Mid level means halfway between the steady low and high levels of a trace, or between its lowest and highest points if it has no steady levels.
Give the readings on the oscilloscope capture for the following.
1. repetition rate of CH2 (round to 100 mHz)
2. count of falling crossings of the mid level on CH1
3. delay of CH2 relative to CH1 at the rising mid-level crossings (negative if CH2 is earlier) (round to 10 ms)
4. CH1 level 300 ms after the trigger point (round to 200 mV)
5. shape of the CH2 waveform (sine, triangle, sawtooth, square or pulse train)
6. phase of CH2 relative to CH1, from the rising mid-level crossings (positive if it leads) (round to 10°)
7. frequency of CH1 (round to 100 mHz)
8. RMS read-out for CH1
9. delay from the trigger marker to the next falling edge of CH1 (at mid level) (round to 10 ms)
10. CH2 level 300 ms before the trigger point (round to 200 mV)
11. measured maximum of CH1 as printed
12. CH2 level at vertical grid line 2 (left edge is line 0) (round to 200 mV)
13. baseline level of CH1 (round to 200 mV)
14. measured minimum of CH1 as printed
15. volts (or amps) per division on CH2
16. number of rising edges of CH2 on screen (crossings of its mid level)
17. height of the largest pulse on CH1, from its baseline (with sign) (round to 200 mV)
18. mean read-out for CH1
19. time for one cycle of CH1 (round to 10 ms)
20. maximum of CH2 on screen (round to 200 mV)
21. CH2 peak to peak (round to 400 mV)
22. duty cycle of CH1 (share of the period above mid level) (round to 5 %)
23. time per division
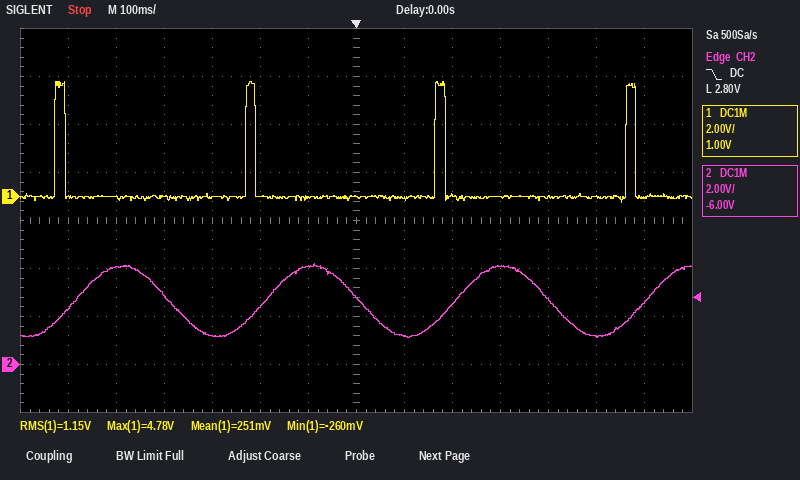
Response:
2.5 Hz
4
+40 ms
0.0 V
sine
-40°
2.5 Hz
1.15 V
190 ms
1.2 V
4.78 V
4.0 V
0.0 V
-260 mV
2 V
4
+4.8 V
251 mV
400 ms
4.2 V
3.2 V
5 %
100 ms
